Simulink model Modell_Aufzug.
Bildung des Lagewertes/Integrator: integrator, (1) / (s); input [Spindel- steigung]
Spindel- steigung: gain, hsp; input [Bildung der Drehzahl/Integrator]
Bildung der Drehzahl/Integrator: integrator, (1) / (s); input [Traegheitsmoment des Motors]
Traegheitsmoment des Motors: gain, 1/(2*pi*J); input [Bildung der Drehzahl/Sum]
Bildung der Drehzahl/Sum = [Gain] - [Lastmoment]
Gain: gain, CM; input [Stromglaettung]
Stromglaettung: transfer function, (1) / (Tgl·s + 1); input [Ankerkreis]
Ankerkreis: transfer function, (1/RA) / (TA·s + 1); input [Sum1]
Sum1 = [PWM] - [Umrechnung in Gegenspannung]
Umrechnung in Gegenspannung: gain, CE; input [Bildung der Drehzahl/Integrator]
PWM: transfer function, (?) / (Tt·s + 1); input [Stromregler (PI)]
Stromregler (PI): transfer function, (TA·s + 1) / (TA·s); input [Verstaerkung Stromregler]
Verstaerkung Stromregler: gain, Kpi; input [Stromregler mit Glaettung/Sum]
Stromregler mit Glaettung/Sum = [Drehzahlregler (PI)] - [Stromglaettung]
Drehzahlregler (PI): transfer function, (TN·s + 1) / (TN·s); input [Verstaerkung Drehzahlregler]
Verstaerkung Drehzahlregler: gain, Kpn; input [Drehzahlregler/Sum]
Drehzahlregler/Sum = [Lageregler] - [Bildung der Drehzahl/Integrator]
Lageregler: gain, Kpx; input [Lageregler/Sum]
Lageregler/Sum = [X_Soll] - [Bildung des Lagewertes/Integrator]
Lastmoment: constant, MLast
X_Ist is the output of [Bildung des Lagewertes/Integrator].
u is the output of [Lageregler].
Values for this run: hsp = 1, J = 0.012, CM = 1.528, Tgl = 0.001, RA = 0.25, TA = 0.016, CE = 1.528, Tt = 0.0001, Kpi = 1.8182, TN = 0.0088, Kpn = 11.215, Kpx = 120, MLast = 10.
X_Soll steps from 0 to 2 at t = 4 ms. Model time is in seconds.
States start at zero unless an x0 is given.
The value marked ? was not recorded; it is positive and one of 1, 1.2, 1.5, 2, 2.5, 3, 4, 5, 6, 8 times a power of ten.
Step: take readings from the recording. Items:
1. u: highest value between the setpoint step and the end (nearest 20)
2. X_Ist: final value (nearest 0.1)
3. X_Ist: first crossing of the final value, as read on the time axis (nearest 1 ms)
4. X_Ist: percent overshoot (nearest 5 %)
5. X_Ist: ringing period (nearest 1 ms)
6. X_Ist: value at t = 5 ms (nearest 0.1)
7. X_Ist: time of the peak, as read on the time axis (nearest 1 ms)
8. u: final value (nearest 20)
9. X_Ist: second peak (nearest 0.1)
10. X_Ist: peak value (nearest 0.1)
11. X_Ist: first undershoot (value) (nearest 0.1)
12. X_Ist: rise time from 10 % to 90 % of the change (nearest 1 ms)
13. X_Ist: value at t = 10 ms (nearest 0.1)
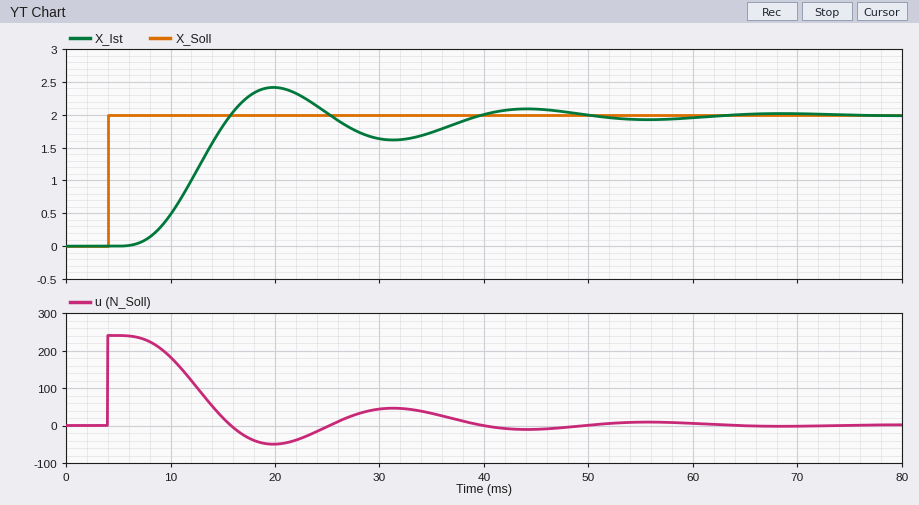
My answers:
240
2.0
16 ms
20 %
24 ms
0.0
20 ms
0
2.1
2.4
1.6
6 ms
0.5
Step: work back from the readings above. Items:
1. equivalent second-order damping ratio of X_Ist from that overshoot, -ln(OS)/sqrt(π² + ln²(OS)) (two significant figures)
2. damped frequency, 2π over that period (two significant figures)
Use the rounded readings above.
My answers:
0.46
0.26 rad/ms
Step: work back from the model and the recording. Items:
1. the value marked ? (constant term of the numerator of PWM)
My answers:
1.2
